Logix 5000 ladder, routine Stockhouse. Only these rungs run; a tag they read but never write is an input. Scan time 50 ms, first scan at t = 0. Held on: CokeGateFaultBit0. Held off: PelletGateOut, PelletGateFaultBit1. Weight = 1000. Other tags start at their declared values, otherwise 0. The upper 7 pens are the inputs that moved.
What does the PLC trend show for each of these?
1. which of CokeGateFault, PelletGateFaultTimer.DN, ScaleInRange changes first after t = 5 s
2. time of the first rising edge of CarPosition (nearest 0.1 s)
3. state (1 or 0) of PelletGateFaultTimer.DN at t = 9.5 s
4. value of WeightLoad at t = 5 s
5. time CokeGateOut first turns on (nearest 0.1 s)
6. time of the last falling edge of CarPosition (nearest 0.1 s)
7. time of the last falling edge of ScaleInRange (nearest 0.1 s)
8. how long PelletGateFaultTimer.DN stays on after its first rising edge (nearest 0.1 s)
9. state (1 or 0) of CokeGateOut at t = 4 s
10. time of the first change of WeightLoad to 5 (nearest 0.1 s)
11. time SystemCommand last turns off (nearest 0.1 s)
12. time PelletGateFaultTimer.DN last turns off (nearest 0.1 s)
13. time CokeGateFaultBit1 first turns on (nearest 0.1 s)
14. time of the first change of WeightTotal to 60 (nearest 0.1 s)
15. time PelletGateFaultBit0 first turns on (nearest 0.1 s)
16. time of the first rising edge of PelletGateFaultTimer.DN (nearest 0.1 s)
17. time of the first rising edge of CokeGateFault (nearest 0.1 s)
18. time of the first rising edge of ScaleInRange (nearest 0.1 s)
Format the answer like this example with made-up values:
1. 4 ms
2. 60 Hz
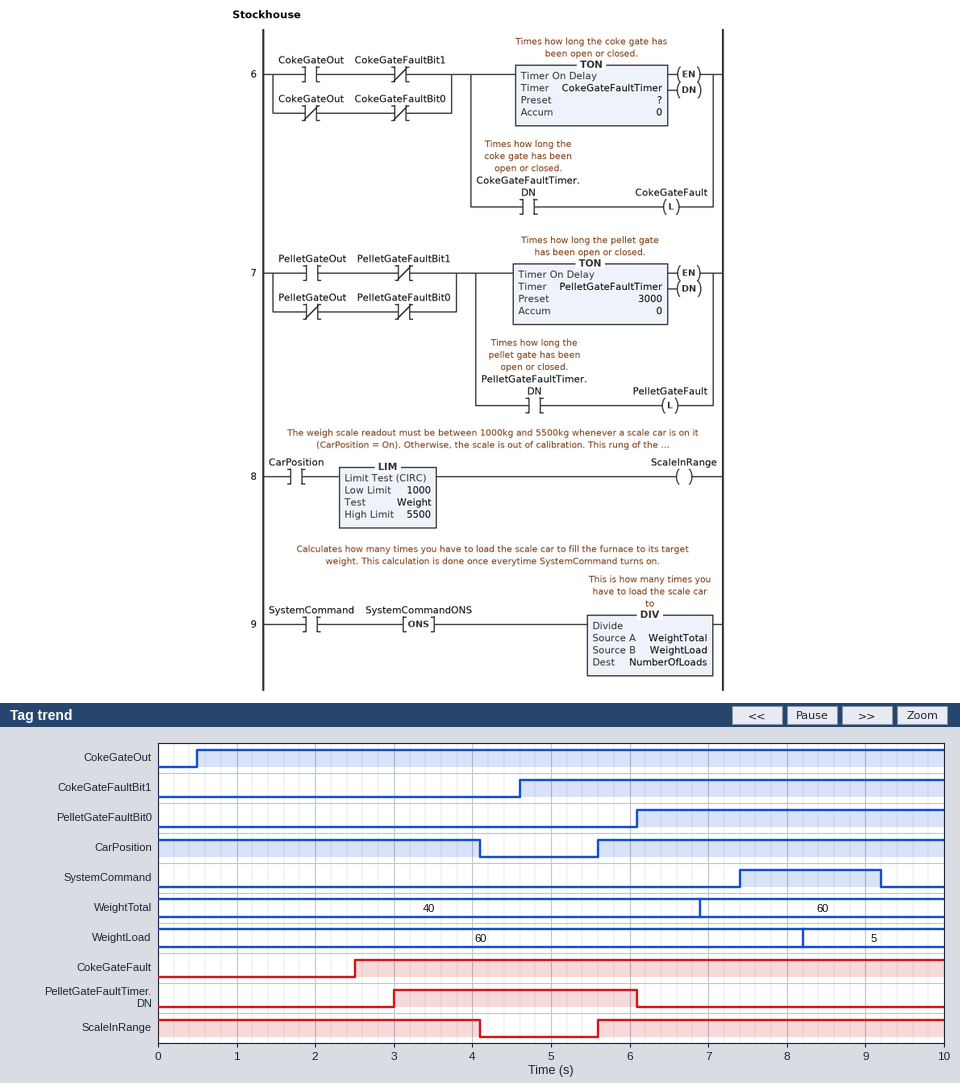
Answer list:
1. ScaleInRange
2. 5.6 s
3. 0
4. 60
5. 0.5 s
6. 4.1 s
7. 4.1 s
8. 3.1 s
9. 1
10. 8.2 s
11. 9.2 s
12. 6.1 s
13. 4.6 s
14. 6.9 s
15. 6.1 s
16. 3.0 s
17. 2.5 s
18. 5.6 s
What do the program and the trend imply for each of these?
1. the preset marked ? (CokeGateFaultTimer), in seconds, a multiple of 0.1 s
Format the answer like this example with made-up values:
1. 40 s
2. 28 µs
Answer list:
1. 2.0 s
